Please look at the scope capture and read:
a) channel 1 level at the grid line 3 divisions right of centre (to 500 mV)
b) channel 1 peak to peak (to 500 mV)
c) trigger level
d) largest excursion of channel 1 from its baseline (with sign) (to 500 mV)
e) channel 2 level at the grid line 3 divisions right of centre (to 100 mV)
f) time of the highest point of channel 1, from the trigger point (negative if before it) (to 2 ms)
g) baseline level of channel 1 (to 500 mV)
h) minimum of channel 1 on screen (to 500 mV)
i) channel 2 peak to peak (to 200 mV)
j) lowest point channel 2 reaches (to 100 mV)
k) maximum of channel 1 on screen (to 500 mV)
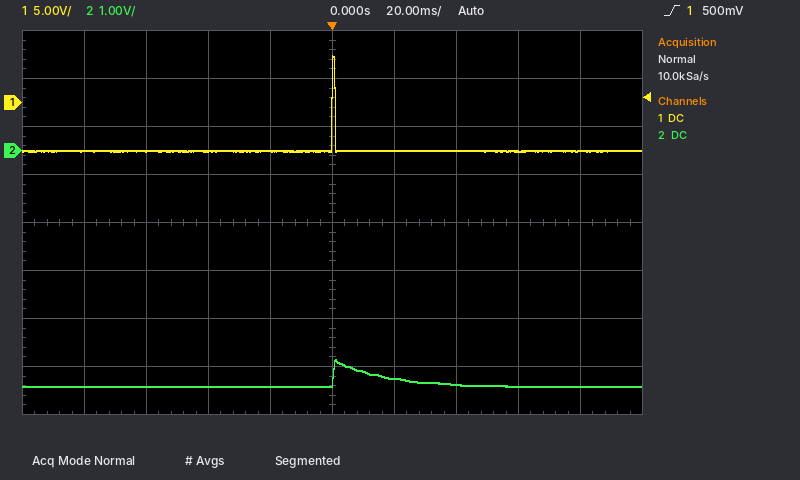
-5.0 V
10.0 V
500 mV
+10.0 V
-4.9 V
0 ms
-5.0 V
-5.0 V
600 mV
-4.9 V
5.0 V
